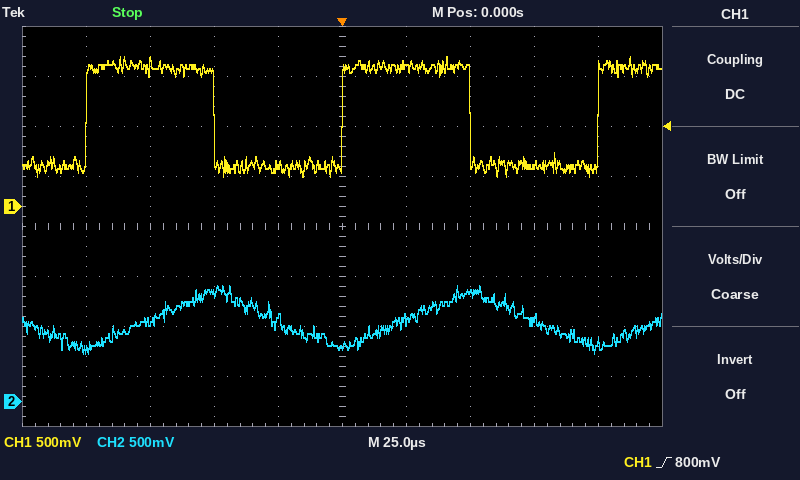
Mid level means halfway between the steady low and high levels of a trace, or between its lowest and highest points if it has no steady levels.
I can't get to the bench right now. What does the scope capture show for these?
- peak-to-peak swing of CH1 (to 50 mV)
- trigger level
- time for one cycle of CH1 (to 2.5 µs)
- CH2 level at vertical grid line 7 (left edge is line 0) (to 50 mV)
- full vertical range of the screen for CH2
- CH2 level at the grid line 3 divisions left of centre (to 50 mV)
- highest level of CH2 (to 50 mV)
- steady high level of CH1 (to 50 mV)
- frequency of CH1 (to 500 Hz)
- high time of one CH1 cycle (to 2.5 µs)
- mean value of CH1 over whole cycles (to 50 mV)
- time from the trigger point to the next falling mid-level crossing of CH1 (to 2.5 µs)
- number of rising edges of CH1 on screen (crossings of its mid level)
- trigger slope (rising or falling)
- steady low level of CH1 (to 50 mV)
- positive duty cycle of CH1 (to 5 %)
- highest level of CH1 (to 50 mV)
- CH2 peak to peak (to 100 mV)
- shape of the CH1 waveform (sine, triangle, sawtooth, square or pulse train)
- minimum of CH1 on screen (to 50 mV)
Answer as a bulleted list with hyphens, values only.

- 1.20 V
- 800 mV
- 100.0 µs
- 1.10 V
- 4 V
- 800 mV
- 1.15 V
- 1.40 V
- 10.0 kHz
- 50.0 µs
- 900 mV
- 50.0 µs
- 3
- rising
- 400 mV
- 50 %
- 1.50 V
- 700 mV
- square
- 300 mV
